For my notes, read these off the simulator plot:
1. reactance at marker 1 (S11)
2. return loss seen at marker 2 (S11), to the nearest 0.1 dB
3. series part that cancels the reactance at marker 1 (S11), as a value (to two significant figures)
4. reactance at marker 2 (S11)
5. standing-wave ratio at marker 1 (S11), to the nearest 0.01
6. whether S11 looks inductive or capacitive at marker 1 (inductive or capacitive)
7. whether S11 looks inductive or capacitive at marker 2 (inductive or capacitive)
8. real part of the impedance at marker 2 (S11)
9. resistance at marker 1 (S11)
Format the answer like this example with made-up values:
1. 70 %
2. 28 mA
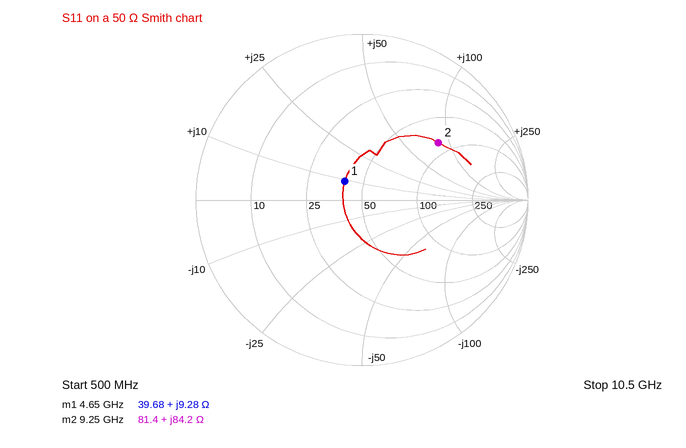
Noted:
1. +9.28 Ω
2. 4.8 dB
3. 3.7 pF
4. +84.2 Ω
5. 1.36
6. inductive
7. inductive
8. 81.4 Ω
9. 39.68 Ω
